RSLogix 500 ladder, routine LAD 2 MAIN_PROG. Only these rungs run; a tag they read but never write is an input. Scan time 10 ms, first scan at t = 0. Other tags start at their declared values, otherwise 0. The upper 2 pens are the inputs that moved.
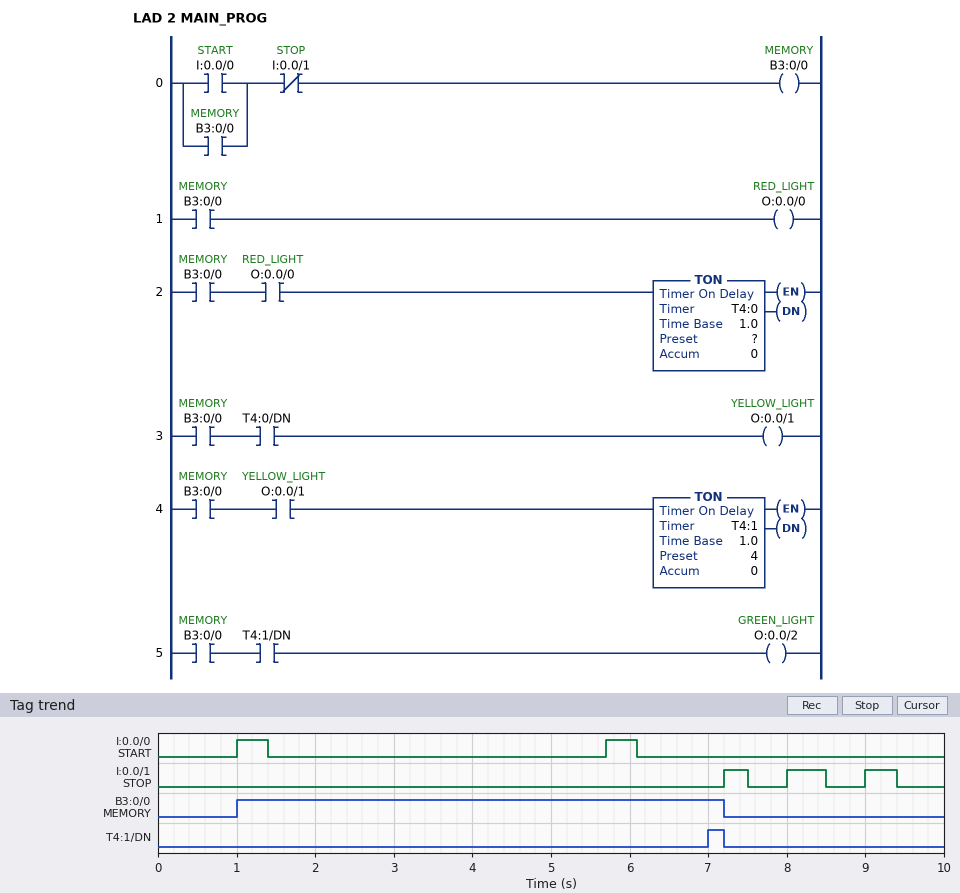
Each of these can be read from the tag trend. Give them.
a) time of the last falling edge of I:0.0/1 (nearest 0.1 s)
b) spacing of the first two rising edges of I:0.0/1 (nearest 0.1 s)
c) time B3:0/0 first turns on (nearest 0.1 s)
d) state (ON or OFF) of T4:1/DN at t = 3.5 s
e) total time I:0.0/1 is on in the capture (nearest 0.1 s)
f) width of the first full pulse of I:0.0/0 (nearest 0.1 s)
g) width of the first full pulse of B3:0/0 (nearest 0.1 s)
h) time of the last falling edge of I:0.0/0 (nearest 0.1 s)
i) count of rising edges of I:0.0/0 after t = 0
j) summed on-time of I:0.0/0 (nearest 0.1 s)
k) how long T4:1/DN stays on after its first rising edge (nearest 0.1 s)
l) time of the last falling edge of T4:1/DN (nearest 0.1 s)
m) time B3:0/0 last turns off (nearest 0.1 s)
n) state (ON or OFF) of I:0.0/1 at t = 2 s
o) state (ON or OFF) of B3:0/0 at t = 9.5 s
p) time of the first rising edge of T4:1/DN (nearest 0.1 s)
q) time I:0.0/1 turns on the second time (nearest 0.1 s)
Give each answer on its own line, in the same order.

9.4 s
0.8 s
1.0 s
OFF
1.2 s
0.4 s
6.2 s
6.1 s
2
0.8 s
0.2 s
7.2 s
7.2 s
OFF
OFF
7.0 s
8.0 s
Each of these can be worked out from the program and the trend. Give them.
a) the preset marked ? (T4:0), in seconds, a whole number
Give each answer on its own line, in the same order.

2 s
